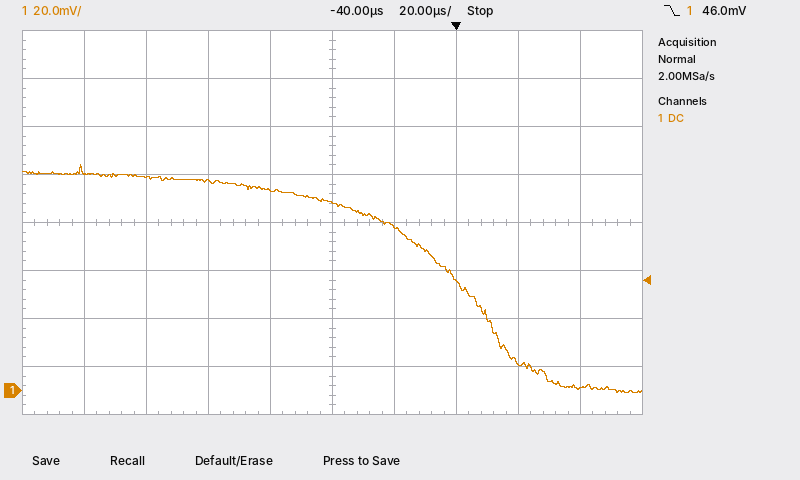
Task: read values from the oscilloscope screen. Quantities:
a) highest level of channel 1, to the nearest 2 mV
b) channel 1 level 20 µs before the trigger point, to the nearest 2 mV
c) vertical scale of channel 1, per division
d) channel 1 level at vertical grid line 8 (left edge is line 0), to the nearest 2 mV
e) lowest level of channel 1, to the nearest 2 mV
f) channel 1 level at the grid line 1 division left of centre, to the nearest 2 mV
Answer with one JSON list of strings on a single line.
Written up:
["94 mV", "68 mV", "20 mV", "12 mV", "0 mV", "84 mV"]
